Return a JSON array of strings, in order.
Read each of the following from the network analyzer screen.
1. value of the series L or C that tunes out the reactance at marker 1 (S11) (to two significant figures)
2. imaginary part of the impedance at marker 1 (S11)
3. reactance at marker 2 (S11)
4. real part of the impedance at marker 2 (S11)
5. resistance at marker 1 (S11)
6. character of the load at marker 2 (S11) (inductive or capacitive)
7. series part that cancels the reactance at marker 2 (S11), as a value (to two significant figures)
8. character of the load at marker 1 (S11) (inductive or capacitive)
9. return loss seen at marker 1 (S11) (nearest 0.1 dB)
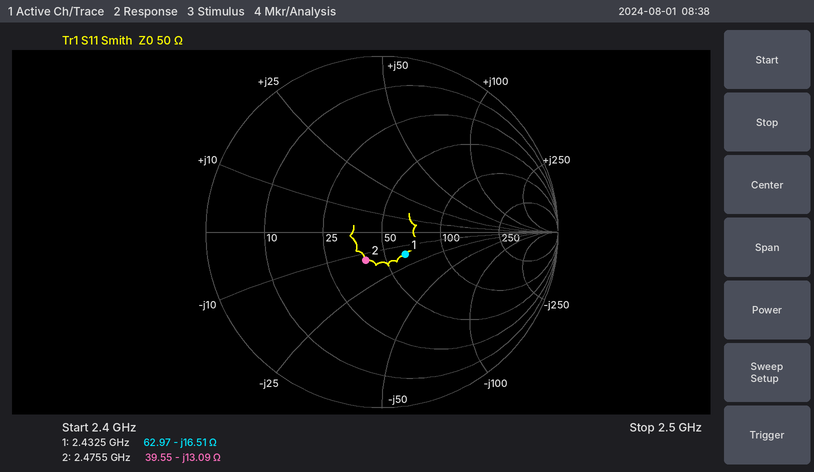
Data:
["1.1 nH", "-16.51 Ω", "-13.09 Ω", "39.55 Ω", "62.97 Ω", "capacitive", "840 pH", "capacitive", "14.7 dB"]
